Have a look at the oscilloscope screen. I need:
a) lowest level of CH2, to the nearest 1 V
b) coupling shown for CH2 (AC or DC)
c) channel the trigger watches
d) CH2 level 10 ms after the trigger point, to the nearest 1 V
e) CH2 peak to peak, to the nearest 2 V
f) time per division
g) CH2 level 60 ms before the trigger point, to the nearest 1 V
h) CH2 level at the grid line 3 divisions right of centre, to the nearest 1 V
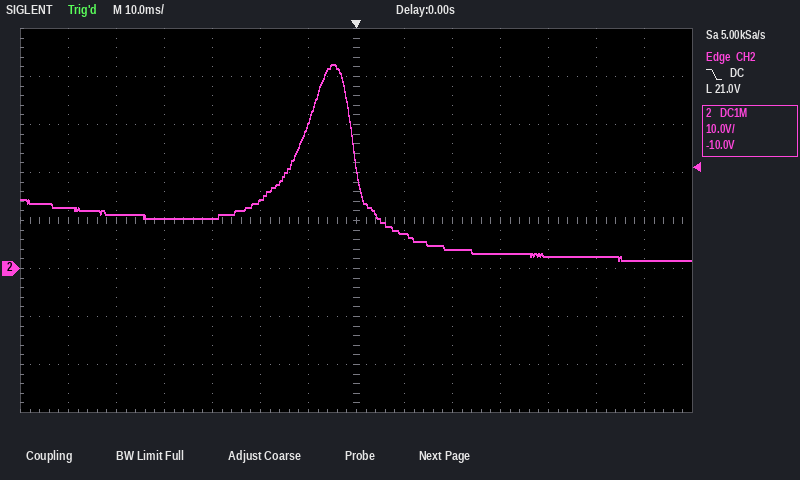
2 V
DC
CH2
7 V
40 V
10 ms
13 V
3 V
